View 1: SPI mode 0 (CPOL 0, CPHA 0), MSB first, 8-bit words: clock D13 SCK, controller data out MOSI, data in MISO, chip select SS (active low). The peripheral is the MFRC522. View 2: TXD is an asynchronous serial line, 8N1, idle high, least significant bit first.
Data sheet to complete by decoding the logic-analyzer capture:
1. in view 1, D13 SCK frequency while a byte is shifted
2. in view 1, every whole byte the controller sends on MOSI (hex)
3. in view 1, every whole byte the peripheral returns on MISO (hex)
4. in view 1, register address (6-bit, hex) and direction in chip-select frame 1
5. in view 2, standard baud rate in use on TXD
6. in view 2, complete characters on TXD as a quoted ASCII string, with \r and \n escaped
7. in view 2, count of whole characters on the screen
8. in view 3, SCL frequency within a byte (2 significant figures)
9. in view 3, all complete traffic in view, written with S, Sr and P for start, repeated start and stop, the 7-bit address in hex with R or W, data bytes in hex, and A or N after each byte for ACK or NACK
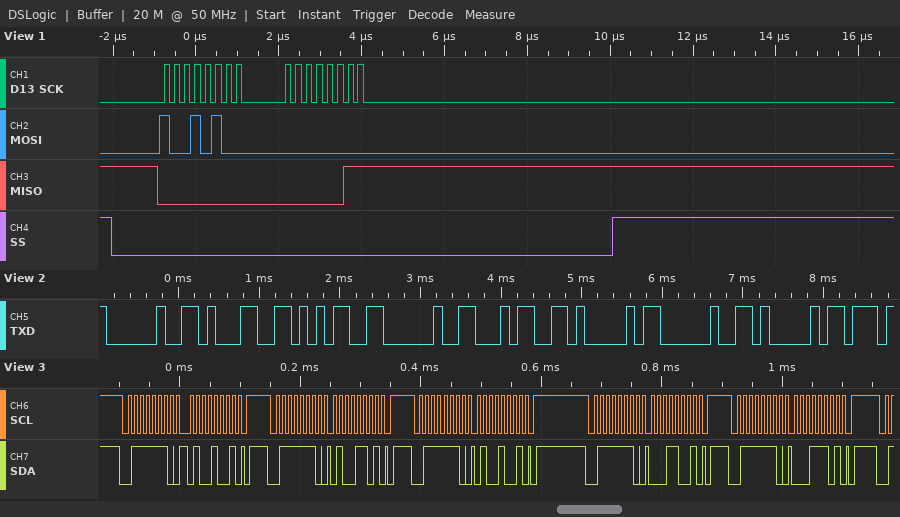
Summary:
4 MHz
94 00
00 03
0x0A read
9600 baud
" 15 4A A"
8
100 kHz
S 3FW A 49 A P S 3FW A 4D A P S 3FW A 49 A P S 3FW A 19 A P S 3FW A 1D A P
